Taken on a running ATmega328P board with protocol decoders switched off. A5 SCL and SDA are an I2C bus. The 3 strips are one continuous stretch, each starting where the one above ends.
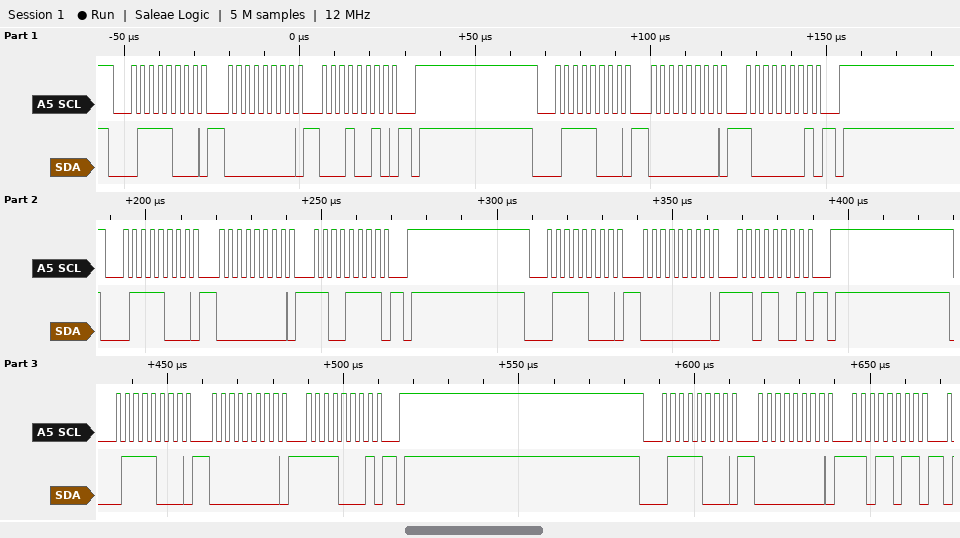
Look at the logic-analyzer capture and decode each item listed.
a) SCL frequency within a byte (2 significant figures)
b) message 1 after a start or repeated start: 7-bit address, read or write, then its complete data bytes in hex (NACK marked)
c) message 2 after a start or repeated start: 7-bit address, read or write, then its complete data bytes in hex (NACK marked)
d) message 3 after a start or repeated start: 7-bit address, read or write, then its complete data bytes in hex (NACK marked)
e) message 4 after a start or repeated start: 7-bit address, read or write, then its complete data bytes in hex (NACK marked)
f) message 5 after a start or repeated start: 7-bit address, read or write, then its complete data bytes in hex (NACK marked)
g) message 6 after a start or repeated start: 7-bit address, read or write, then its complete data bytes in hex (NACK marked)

400 kHz
0x3C write: 00 12
0x3C write: 00 81
0x3C write: 00 CF
0x3C write: 00 D9
0x3C write: 00 F1
0x3C write: 00 DB
